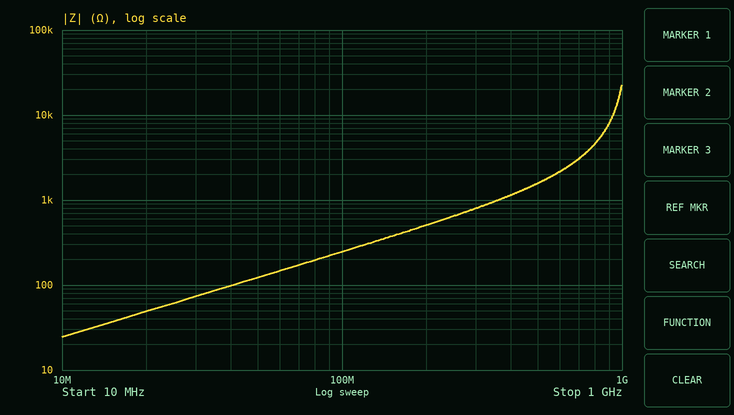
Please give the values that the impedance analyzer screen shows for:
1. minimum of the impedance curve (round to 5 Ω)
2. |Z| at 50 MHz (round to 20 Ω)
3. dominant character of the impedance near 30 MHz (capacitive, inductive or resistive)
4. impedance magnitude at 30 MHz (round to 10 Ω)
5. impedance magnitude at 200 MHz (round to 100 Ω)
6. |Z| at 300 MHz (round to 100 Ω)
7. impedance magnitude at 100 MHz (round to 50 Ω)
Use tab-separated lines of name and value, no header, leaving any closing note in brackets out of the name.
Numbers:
minimum of the impedance curve	25 Ω
|Z| at 50 MHz	120 Ω
dominant character of the impedance near 30 MHz	inductive
impedance magnitude at 30 MHz	70 Ω
impedance magnitude at 200 MHz	500 Ω
|Z| at 300 MHz	800 Ω
impedance magnitude at 100 MHz	250 Ω
